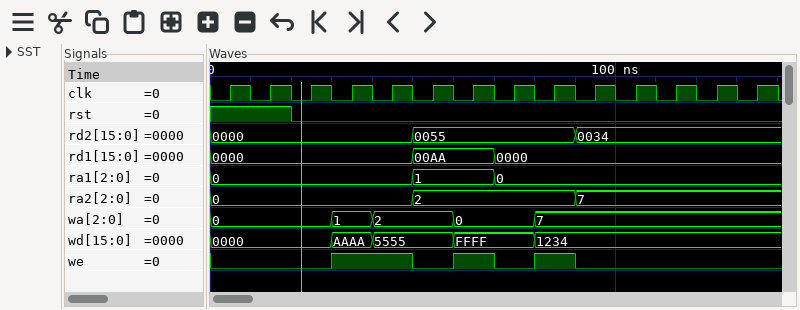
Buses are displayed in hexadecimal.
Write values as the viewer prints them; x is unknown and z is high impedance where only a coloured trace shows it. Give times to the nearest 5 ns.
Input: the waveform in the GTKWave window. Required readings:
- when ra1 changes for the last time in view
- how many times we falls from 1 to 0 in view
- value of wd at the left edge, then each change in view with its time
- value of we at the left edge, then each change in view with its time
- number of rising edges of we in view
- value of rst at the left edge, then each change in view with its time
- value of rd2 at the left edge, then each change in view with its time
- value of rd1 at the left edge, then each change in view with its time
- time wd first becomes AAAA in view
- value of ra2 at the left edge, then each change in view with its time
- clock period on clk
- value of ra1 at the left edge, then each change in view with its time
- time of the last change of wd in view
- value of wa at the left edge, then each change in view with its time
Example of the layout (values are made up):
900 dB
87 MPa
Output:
70 ns
3
0000, AAAA at 30 ns, 5555 at 40 ns, FFFF at 60 ns, 1234 at 80 ns
0, 1 at 30 ns, 0 at 50 ns, 1 at 60 ns, 0 at 70 ns, 1 at 80 ns, 0 at 90 ns
3
1, 0 at 20 ns
0000, 0055 at 50 ns, 0034 at 90 ns
0000, 00AA at 50 ns, 0000 at 70 ns
30 ns
0, 2 at 50 ns, 7 at 90 ns
10 ns
0, 1 at 50 ns, 0 at 70 ns
80 ns
0, 1 at 30 ns, 2 at 40 ns, 0 at 60 ns, 7 at 80 ns
